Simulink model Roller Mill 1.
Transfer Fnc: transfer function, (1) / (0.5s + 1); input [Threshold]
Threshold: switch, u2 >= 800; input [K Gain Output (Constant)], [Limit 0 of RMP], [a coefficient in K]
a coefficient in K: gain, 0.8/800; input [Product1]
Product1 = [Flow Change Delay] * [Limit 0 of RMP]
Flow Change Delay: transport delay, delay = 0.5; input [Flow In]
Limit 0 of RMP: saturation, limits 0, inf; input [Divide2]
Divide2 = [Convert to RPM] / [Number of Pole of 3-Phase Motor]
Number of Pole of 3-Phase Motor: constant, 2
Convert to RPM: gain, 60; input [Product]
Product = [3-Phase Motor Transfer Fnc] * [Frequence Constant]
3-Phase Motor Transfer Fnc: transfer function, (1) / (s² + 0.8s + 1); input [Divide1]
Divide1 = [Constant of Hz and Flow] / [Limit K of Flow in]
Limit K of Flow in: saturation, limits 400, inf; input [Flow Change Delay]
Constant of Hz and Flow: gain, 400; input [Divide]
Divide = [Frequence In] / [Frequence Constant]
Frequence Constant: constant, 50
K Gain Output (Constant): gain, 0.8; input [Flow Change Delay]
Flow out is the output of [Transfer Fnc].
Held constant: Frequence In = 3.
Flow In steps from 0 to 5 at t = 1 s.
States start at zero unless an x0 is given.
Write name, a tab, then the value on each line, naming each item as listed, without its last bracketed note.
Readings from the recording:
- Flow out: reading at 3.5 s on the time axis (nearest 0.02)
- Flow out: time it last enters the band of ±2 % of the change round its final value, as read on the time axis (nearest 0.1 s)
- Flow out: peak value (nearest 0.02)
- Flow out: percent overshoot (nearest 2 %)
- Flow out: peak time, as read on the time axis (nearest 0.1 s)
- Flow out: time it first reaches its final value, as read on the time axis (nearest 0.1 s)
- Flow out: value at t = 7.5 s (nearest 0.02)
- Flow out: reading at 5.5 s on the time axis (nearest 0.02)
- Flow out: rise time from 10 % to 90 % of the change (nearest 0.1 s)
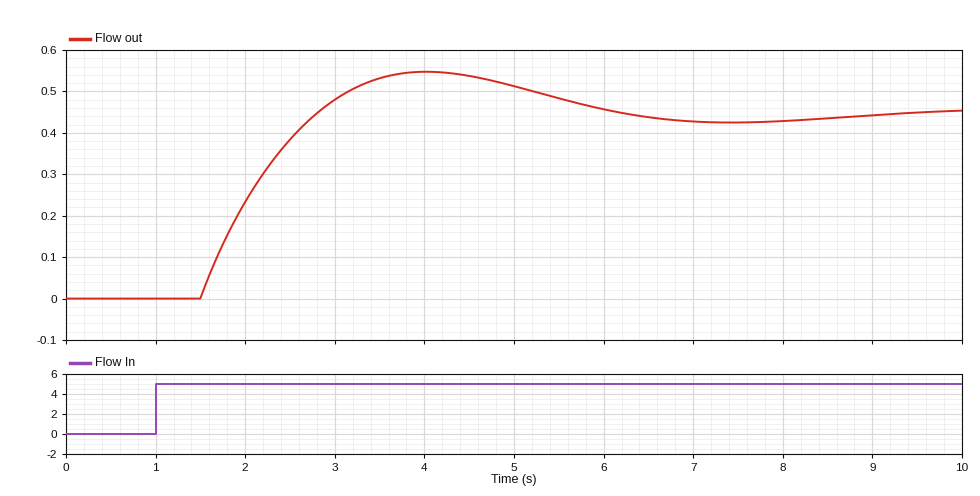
Flow out: reading at 3.5 s on the time axis	0.54
Flow out: time it last enters the band of ±2 % of the change round its final value, as read on the time axis	8.9 s
Flow out: peak value	0.54
Flow out: percent overshoot	22 %
Flow out: peak time, as read on the time axis	4.0 s
Flow out: time it first reaches its final value, as read on the time axis	2.8 s
Flow out: value at t = 7.5 s	0.42
Flow out: reading at 5.5 s on the time axis	0.48
Flow out: rise time from 10 % to 90 % of the change	1.0 s
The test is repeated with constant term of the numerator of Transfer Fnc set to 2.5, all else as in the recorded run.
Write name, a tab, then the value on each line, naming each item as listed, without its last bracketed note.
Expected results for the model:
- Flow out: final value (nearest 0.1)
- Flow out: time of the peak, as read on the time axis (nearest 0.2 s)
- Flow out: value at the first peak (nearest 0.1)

Flow out: final value	1.1
Flow out: time of the peak, as read on the time axis	4.0 s
Flow out: value at the first peak	1.4
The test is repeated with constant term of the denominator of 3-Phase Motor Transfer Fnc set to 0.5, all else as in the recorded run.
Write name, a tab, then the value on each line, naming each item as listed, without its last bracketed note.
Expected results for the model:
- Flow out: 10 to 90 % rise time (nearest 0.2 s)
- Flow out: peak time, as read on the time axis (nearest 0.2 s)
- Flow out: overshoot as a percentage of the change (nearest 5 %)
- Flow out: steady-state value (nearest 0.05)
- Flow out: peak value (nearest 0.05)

Flow out: 10 to 90 % rise time	2.2 s
Flow out: peak time, as read on the time axis	6.0 s
Flow out: overshoot as a percentage of the change	10 %
Flow out: steady-state value	0.90
Flow out: peak value	1.00
